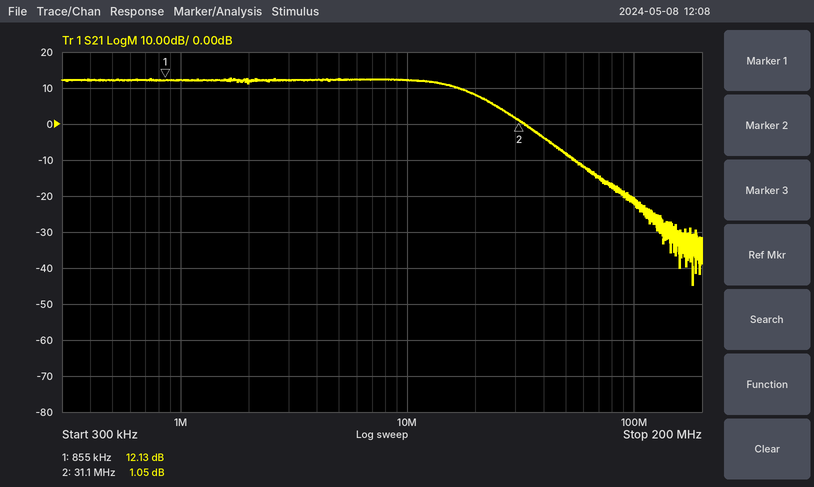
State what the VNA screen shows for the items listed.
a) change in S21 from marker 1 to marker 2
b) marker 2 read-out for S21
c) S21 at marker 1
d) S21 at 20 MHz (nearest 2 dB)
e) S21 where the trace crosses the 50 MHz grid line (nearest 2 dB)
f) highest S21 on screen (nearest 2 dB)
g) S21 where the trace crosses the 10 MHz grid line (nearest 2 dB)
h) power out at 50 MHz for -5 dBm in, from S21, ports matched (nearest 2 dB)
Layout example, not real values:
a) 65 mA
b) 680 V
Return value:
a) -11.08 dB
b) 1.05 dB
c) 12.13 dB
d) 8 dB
e) -8 dB
f) 12 dB
g) 12 dB
h) -14 dBm
